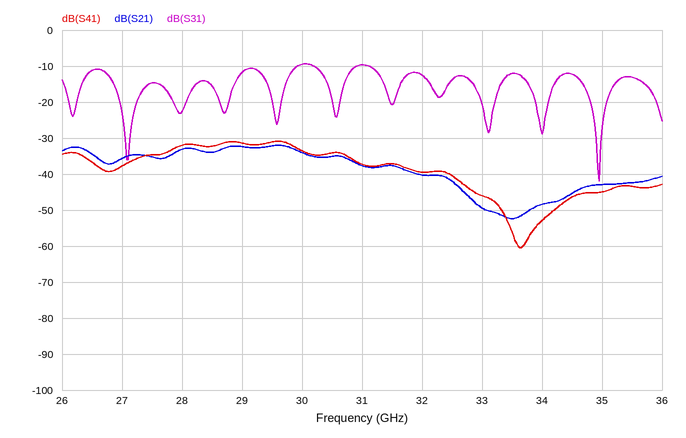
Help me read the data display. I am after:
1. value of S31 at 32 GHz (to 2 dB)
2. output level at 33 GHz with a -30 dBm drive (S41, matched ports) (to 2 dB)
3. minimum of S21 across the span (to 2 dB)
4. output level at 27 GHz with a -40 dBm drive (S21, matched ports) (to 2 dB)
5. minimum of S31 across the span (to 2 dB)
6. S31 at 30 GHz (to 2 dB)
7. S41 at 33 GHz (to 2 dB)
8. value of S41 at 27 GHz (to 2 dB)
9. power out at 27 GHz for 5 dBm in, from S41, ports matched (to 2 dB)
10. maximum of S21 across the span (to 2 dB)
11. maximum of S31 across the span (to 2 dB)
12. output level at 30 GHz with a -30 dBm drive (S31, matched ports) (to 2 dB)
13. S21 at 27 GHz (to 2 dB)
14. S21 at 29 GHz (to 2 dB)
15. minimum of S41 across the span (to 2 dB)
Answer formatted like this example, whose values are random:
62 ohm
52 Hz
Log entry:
-12 dB
-76 dBm
-52 dB
-76 dBm
-42 dB
-10 dB
-46 dB
-38 dB
-32 dBm
-32 dB
-10 dB
-40 dBm
-36 dB
-32 dB
-60 dB
